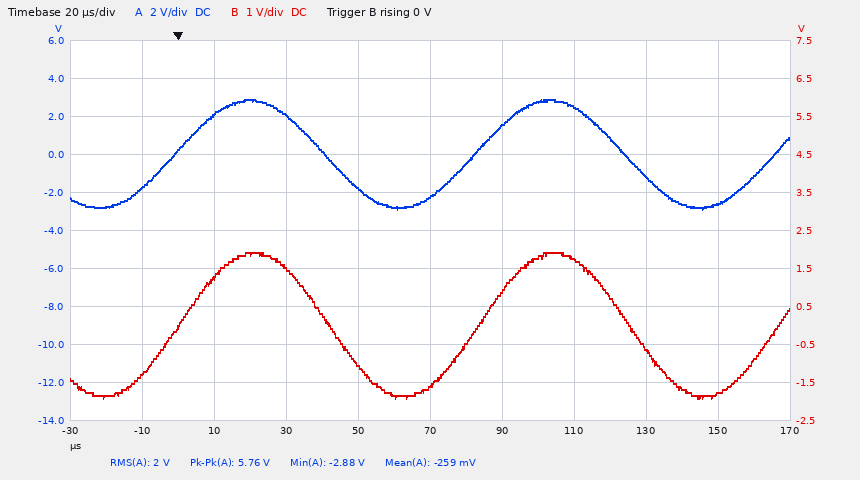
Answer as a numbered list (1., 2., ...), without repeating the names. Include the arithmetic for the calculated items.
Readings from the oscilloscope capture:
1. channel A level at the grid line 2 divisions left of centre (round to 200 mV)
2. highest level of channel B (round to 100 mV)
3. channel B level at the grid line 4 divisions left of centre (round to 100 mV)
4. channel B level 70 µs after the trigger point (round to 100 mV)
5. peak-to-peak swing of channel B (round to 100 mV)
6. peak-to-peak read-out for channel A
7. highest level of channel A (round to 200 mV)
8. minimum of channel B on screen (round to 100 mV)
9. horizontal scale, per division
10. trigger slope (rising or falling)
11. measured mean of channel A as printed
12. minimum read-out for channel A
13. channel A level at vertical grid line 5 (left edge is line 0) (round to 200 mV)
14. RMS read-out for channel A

1. 2.0 V
2. 1.9 V
3. -1.3 V
4. -1.6 V
5. 1.9 V − (-1.9 V) = 3.8 V
6. 5.76 V
7. 2.8 V
8. -1.9 V
9. 20 µs
10. rising
11. -259 mV
12. -2.88 V
13. -2.2 V
14. 2 V
